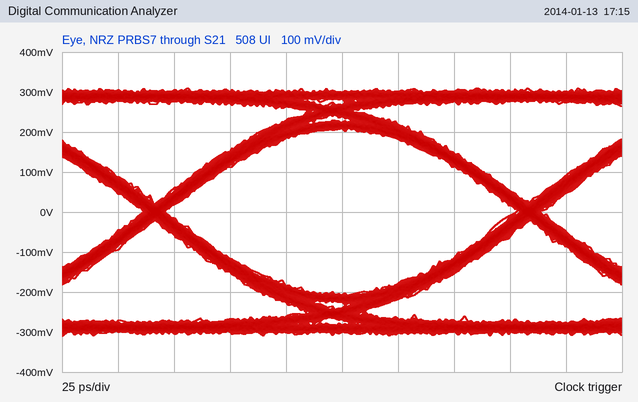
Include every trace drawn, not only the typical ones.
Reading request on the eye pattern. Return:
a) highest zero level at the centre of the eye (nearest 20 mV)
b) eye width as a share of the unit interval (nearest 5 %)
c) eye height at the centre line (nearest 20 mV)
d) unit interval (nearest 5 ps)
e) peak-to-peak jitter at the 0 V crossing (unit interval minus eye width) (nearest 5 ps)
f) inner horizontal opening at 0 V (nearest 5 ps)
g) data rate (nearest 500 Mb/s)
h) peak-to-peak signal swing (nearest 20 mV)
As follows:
-200 mV
95 %
420 mV
165 ps
10 ps
155 ps
6.0 Gb/s
620 mV
